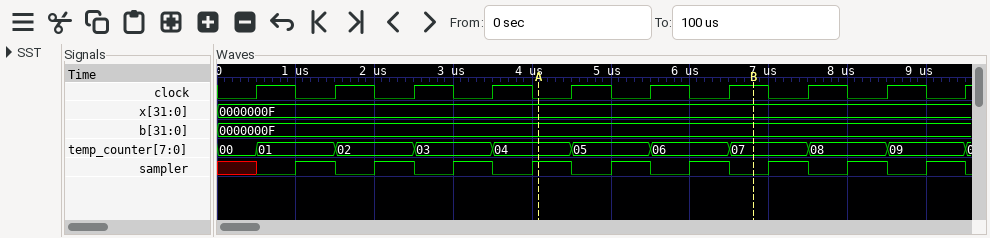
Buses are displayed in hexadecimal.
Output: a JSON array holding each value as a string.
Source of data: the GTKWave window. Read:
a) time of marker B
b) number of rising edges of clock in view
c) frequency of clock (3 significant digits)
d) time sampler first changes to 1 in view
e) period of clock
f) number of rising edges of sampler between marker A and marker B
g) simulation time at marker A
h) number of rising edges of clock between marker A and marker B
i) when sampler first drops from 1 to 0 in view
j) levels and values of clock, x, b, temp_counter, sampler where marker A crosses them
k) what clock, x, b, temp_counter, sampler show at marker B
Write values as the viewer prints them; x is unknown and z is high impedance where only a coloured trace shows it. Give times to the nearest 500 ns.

["7000 ns", "10", "1.00 MHz", "1000 ns", "1000 ns", "2", "4000 ns", "3", "1500 ns", "clock=0, x=0000000F, b=0000000F, temp_counter=04, sampler=1", "clock=1, x=0000000F, b=0000000F, temp_counter=07, sampler=0"]
